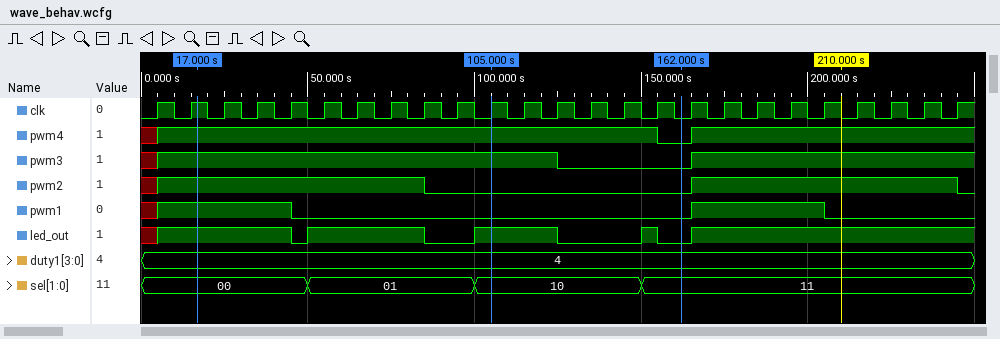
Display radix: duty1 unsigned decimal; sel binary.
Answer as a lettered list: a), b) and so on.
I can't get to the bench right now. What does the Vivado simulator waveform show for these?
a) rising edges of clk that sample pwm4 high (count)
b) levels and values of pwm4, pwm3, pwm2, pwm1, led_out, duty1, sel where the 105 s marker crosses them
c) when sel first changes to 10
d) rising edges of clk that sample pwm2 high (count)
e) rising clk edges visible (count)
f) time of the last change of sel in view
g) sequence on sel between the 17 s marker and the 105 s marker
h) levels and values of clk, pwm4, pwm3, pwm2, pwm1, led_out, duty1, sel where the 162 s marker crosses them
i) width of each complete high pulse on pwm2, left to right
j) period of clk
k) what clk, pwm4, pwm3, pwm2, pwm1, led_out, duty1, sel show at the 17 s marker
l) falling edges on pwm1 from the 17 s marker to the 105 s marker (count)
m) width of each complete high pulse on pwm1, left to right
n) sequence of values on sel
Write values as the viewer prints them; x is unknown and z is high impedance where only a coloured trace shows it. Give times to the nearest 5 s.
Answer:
a) 23
b) pwm4=1, pwm3=1, pwm2=0, pwm1=0, led_out=1, duty1=4, sel=10
c) 100 s
d) 16
e) 25
f) 150 s
g) 00, 01, 10
h) clk=0, pwm4=0, pwm3=0, pwm2=0, pwm1=0, led_out=0, duty1=4, sel=11
i) 80 s
j) 10 s
k) clk=1, pwm4=1, pwm3=1, pwm2=1, pwm1=1, led_out=1, duty1=4, sel=00
l) 1
m) 40 s
n) 00, 01, 10, 11
